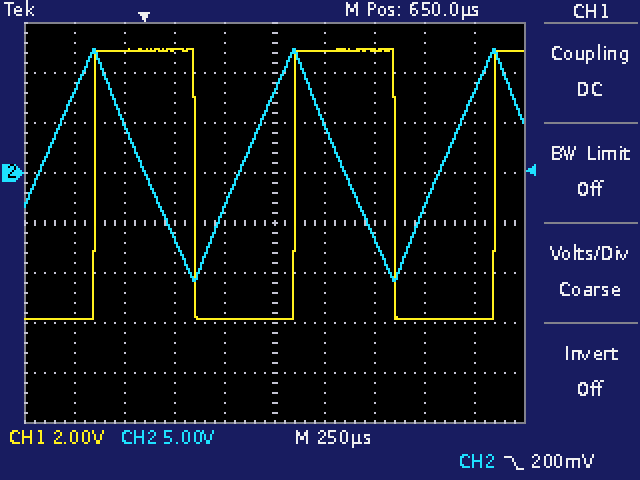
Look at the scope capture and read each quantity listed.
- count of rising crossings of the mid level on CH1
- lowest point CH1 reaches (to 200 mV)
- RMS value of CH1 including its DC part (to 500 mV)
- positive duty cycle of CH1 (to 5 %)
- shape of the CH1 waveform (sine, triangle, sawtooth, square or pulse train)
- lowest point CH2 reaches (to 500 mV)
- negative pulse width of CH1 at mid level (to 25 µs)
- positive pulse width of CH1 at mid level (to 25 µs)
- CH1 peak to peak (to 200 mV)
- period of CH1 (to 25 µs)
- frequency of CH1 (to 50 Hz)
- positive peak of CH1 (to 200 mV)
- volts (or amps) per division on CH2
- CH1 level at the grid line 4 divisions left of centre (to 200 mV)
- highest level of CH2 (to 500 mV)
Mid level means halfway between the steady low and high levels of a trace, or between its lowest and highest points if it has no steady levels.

3
-5.8 V
5.5 V
50 %
square
-11.0 V
500 µs
500 µs
10.8 V
1.000 ms
1.00 kHz
5.0 V
5 V
-5.8 V
12.5 V
